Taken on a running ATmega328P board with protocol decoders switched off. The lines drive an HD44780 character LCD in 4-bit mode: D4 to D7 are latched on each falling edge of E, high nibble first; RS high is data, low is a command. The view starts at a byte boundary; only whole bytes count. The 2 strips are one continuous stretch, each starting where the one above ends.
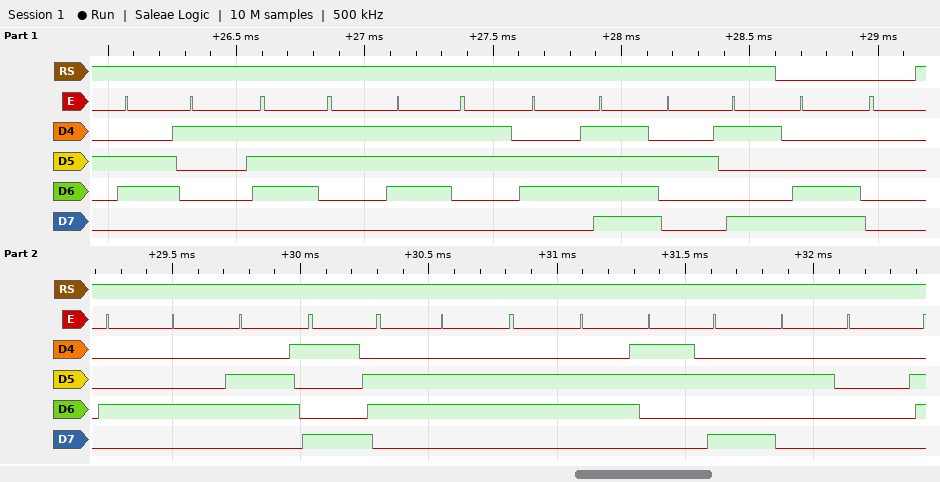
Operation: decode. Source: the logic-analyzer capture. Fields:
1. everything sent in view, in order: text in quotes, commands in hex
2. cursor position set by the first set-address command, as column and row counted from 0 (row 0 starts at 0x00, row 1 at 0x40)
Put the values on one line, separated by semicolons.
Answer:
"asso)" 0xC0 "Diff: "; column 0, row 1
